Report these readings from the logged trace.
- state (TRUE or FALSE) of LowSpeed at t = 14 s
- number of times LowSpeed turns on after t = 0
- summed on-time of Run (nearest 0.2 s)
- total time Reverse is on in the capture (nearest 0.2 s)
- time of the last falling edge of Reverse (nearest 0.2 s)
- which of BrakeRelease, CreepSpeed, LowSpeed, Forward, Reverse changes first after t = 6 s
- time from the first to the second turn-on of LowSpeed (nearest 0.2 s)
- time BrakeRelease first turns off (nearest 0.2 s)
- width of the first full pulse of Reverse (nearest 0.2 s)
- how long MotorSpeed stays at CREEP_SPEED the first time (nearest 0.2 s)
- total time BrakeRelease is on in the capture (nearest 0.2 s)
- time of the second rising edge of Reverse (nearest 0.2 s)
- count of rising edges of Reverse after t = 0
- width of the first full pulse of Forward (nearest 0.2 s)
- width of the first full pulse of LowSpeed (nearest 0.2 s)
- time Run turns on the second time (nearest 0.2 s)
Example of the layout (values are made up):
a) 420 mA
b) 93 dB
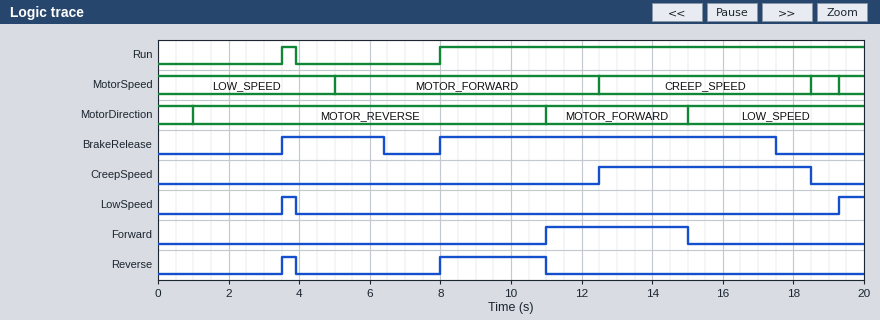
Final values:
a) FALSE
b) 2
c) 12.4 s
d) 3.4 s
e) 11.0 s
f) BrakeRelease
g) 15.8 s
h) 6.4 s
i) 0.4 s
j) 6.0 s
k) 12.4 s
l) 8.0 s
m) 2
n) 4.0 s
o) 0.4 s
p) 8.0 s
